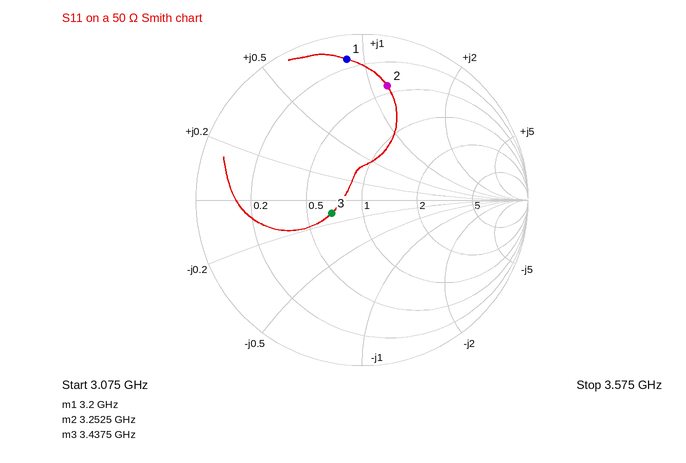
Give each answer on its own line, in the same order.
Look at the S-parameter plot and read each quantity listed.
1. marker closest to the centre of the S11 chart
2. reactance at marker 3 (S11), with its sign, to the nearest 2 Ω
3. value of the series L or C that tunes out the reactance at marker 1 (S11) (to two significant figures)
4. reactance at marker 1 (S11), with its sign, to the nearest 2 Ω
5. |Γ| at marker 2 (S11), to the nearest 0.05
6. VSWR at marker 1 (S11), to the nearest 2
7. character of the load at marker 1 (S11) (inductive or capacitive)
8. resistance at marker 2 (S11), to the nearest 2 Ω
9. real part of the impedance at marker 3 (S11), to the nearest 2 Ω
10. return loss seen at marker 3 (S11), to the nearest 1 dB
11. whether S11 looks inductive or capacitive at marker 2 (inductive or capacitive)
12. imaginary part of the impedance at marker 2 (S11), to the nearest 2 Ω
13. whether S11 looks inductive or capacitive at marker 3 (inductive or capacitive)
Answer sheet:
marker 3
-6 Ω
1.1 pF
+44 Ω
0.70
12
inductive
22 Ω
34 Ω
14 dB
inductive
+58 Ω
capacitive
